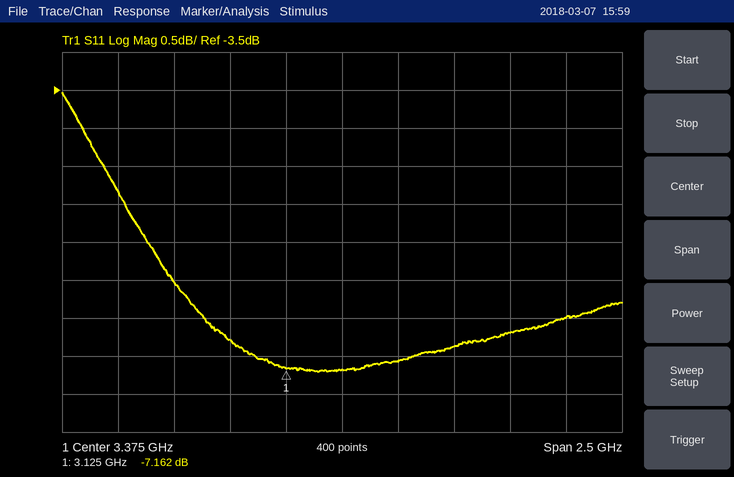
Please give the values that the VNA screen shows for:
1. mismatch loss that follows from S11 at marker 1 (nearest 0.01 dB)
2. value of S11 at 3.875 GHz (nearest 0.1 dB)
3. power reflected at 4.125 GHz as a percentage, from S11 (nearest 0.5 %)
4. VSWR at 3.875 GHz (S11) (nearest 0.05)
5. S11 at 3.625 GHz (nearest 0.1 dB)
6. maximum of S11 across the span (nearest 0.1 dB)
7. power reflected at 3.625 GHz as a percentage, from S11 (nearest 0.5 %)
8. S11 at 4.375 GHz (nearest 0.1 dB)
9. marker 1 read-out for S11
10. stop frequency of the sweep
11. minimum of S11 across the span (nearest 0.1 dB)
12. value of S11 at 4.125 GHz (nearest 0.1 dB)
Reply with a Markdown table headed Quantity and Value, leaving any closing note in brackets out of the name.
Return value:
| Quantity | Value |
|---|---|
| mismatch loss that follows from S11 at marker 1 | 0.93 dB |
| value of S11 at 3.875 GHz | -6.9 dB |
| power reflected at 4.125 GHz as a percentage, from S11 | 21.5 % |
| VSWR at 3.875 GHz (S11) | 2.65 |
| S11 at 3.625 GHz | -7.1 dB |
| maximum of S11 across the span | -3.5 dB |
| power reflected at 3.625 GHz as a percentage, from S11 | 19.5 % |
| S11 at 4.375 GHz | -6.5 dB |
| marker 1 read-out for S11 | -7.162 dB |
| stop frequency of the sweep | 4.625 GHz |
| minimum of S11 across the span | -7.2 dB |
| value of S11 at 4.125 GHz | -6.7 dB |
